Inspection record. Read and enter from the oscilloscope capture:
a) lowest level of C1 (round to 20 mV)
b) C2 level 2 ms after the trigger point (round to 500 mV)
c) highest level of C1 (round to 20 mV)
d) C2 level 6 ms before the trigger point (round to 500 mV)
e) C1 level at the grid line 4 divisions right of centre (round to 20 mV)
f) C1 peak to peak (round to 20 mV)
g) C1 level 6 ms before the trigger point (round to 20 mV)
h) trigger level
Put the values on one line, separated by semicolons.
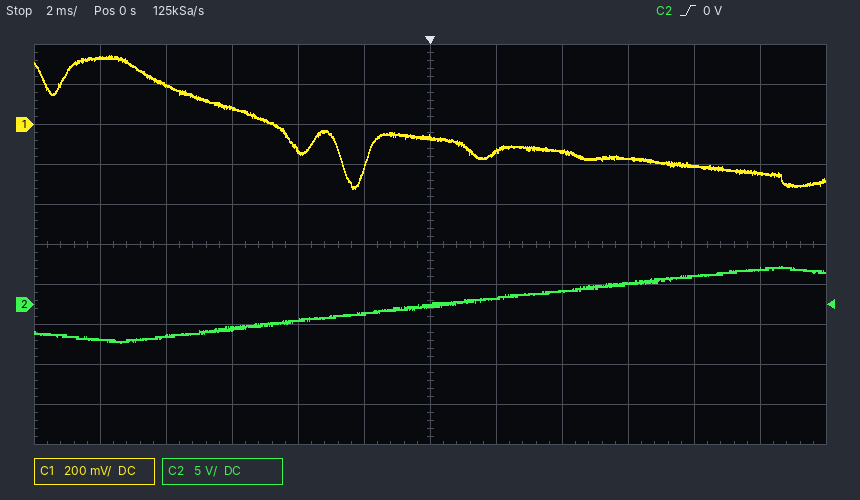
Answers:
-320 mV; 1.0 V; 340 mV; -3.0 V; -200 mV; 660 mV; 80 mV; 0 V
